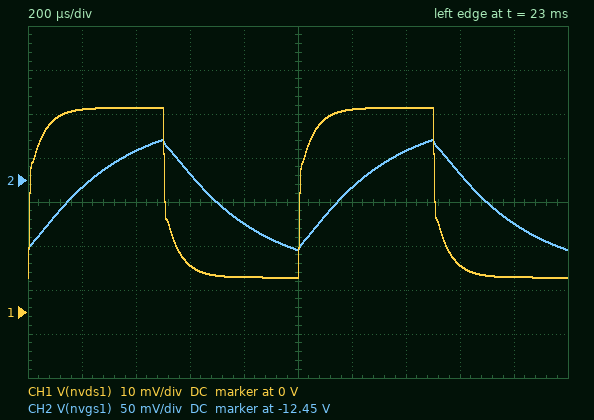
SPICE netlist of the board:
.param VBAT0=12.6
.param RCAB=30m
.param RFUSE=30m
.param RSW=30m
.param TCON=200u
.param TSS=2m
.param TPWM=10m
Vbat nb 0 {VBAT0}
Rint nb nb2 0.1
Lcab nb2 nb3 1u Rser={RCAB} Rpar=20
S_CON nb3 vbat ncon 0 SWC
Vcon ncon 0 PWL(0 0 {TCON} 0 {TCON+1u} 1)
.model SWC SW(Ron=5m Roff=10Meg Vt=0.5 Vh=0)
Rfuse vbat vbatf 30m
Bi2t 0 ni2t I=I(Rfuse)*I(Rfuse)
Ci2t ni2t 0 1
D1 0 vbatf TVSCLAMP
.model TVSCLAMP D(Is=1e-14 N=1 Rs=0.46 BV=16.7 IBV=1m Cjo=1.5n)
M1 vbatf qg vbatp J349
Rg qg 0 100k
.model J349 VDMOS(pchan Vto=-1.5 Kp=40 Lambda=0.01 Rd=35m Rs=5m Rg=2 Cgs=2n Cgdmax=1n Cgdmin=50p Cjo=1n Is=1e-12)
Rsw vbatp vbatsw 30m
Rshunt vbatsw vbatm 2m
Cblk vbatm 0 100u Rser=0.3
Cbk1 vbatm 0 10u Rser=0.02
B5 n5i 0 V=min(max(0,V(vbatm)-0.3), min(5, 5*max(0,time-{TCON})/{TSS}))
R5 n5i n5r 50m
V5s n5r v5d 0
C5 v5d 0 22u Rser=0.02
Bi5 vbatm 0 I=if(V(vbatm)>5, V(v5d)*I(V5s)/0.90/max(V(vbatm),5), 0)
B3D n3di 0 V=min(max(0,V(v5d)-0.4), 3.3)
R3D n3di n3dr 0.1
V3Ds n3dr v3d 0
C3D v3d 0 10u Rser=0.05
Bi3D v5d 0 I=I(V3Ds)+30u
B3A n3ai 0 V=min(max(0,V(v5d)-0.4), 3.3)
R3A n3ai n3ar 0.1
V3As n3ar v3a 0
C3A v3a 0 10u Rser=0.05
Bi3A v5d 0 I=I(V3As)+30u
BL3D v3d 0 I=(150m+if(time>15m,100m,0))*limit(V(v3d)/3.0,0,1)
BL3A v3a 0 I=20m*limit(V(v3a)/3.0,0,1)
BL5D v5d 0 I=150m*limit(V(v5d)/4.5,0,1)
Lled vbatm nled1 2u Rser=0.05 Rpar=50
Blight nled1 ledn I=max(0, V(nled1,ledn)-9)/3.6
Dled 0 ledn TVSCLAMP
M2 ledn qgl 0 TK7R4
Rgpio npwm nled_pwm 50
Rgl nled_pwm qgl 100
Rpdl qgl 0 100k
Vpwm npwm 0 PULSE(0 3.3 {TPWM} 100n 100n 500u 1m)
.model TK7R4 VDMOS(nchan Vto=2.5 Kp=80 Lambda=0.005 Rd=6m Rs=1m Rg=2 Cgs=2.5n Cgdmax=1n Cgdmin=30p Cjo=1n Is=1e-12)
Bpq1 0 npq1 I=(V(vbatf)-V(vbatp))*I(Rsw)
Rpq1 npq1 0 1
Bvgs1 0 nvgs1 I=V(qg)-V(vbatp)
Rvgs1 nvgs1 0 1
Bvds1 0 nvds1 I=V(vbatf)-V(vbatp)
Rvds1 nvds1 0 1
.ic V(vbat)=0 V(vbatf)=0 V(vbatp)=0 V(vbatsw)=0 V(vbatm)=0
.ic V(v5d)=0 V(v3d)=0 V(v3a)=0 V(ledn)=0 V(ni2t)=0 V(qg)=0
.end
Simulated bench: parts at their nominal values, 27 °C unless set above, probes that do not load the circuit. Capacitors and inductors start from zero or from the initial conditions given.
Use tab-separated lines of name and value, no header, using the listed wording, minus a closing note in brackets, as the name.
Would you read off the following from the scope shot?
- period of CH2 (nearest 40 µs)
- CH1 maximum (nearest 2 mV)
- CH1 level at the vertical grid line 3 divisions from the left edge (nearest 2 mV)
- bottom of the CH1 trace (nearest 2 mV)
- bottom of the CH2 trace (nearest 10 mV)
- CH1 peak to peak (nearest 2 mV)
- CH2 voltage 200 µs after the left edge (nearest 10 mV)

period of CH2	1.00 ms
CH1 maximum	46 mV
CH1 level at the vertical grid line 3 divisions from the left edge	10 mV
bottom of the CH1 trace	8 mV
bottom of the CH2 trace	-12.53 V
CH1 peak to peak	38 mV
CH2 voltage 200 µs after the left edge	-12.46 V
